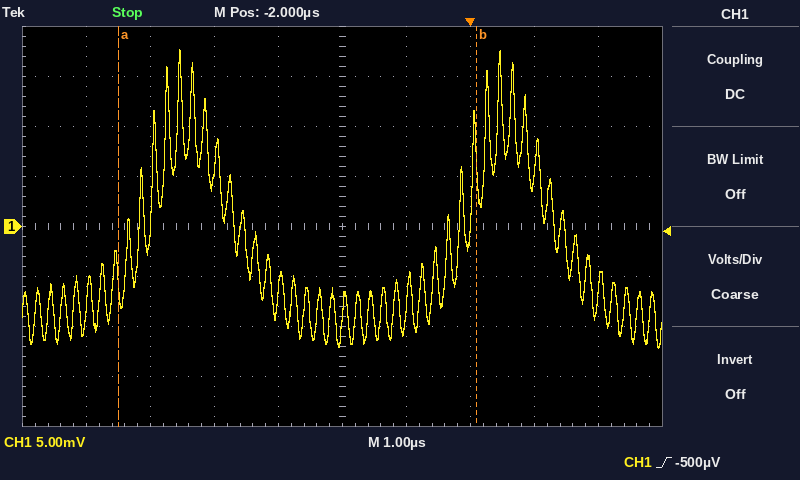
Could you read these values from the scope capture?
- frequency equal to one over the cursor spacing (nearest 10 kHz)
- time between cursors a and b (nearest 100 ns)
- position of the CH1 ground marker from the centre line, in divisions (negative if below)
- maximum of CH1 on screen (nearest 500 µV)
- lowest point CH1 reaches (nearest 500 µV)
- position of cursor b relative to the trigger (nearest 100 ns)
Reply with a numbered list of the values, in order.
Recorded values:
1. 180 kHz
2. 5.6 µs
3. 0.0 div
4. 17.5 mV
5. -12.0 mV
6. +100 ns
